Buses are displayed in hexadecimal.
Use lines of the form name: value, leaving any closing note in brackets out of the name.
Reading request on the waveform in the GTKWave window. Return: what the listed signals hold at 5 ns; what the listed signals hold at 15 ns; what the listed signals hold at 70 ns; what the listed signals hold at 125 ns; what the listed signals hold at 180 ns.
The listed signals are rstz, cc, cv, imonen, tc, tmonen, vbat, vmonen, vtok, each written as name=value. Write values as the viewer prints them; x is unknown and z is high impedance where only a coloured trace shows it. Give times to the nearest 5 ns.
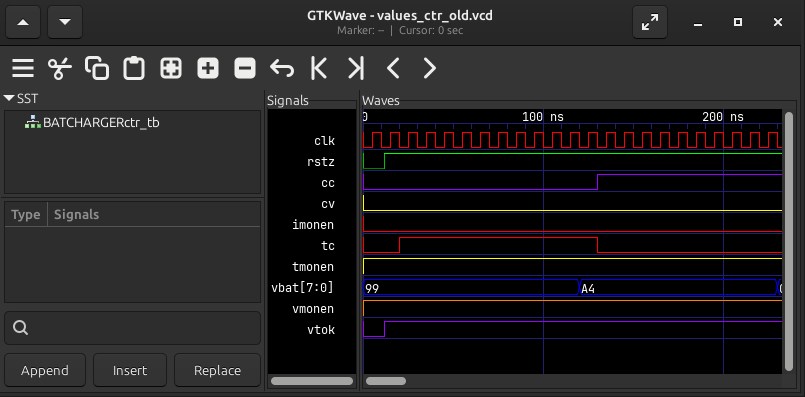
what the listed signals hold at 5 ns: rstz=0, cc=0, cv=0, imonen=0, tc=0, tmonen=1, vbat=99, vmonen=1, vtok=0
what the listed signals hold at 15 ns: rstz=1, cc=0, cv=0, imonen=0, tc=0, tmonen=1, vbat=99, vmonen=1, vtok=1
what the listed signals hold at 70 ns: rstz=1, cc=0, cv=0, imonen=0, tc=1, tmonen=1, vbat=99, vmonen=1, vtok=1
what the listed signals hold at 125 ns: rstz=1, cc=0, cv=0, imonen=0, tc=1, tmonen=1, vbat=A4, vmonen=1, vtok=1
what the listed signals hold at 180 ns: rstz=1, cc=1, cv=0, imonen=0, tc=0, tmonen=1, vbat=A4, vmonen=1, vtok=1
